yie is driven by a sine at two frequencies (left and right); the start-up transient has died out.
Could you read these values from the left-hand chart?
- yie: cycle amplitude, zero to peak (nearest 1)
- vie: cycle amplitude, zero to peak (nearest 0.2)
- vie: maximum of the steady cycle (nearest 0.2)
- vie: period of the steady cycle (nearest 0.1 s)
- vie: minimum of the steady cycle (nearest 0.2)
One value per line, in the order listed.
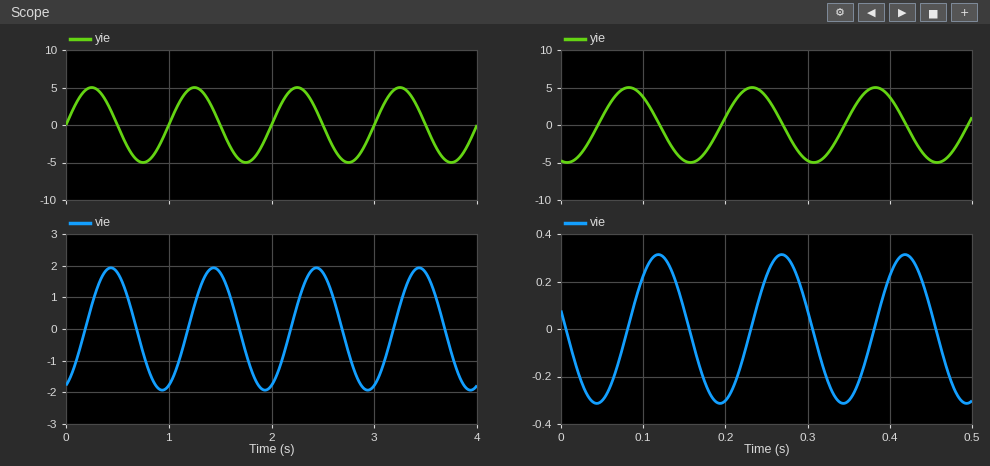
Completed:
5
2.0
2.0
1.0 s
-2.0
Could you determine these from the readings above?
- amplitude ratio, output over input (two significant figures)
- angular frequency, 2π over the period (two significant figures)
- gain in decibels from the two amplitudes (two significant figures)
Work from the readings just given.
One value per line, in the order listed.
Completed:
0.40
6.3 rad/s
-8.0 dB
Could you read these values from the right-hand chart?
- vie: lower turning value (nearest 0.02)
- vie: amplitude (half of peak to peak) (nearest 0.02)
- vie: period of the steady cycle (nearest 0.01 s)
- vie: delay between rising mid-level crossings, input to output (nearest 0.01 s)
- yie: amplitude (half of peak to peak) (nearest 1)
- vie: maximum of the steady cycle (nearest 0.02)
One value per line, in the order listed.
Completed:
-0.32
0.32
0.15 s
0.04 s
5
0.32
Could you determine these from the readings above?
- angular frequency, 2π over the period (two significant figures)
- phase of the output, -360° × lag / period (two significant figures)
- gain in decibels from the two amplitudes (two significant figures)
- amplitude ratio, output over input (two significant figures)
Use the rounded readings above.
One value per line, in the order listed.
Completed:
42 rad/s
-96°
-24 dB
0.064
